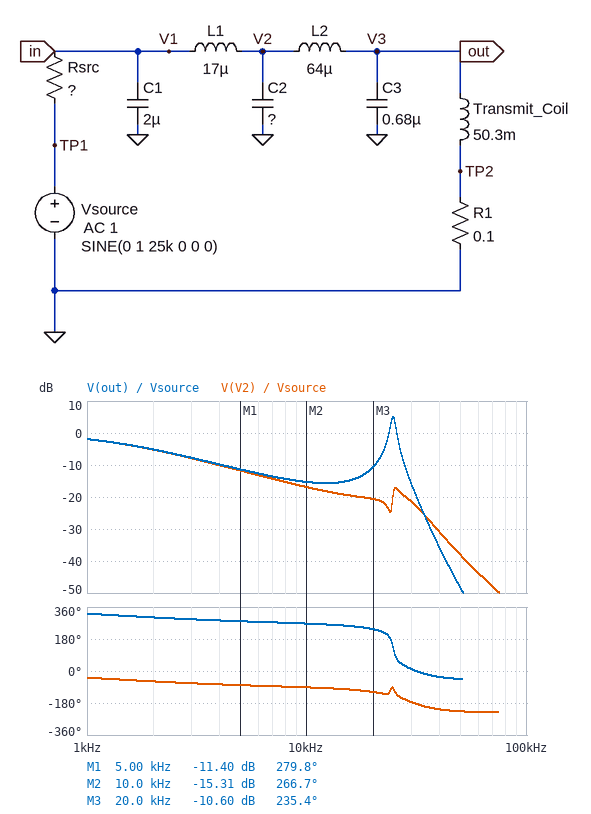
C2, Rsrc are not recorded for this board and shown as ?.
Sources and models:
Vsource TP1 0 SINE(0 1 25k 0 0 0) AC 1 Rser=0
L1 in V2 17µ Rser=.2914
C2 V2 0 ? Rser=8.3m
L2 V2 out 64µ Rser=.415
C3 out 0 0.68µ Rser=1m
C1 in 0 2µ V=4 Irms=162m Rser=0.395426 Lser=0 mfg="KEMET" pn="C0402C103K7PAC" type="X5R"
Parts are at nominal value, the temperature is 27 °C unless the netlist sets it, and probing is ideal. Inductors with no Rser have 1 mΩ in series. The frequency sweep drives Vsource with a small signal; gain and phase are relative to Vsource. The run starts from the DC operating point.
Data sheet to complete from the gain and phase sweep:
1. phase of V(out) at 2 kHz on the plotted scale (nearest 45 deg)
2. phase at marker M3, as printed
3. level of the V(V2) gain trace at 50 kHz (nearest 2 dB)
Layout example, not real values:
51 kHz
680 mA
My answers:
315 deg
235.4 deg
-38 dB
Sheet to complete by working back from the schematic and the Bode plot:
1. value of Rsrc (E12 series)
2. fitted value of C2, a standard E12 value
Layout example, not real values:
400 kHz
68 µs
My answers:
6.8 Ω
15 µF
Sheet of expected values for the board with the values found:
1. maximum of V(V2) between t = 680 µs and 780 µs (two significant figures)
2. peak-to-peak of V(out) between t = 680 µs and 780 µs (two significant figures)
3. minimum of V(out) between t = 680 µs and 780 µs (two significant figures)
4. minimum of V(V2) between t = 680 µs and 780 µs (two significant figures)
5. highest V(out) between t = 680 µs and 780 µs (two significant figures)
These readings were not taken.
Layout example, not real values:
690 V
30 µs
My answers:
130 mV
3.2 V
-1.6 V
-130 mV
1.6 V
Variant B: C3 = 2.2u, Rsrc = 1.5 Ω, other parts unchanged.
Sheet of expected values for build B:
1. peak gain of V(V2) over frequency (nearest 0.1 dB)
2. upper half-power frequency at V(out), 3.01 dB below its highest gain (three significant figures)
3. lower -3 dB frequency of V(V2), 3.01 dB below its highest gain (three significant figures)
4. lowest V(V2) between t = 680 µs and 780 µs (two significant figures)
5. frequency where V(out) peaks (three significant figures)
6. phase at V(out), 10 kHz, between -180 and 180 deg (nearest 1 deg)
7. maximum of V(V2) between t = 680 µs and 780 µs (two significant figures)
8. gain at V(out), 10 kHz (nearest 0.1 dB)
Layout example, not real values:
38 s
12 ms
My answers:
0 dB
15.2 kHz
6.91 Hz
-170 mV
14.4 kHz
-106 deg
170 mV
-0.1 dB
